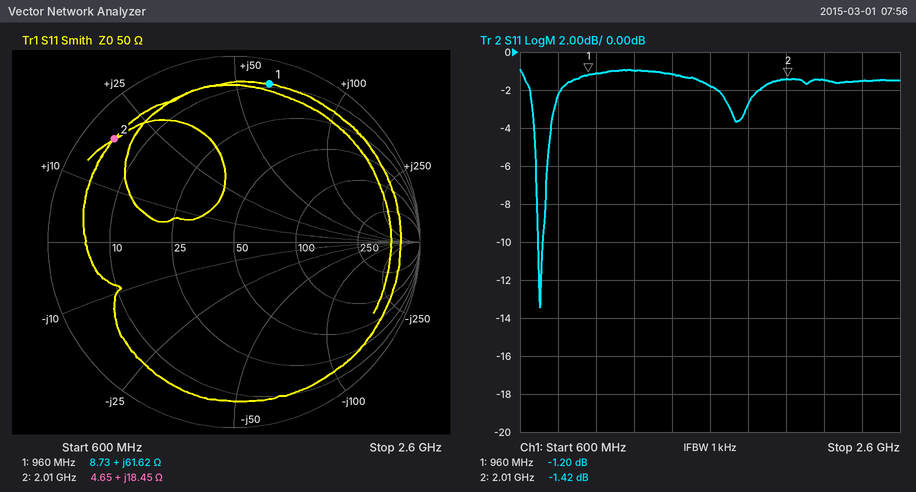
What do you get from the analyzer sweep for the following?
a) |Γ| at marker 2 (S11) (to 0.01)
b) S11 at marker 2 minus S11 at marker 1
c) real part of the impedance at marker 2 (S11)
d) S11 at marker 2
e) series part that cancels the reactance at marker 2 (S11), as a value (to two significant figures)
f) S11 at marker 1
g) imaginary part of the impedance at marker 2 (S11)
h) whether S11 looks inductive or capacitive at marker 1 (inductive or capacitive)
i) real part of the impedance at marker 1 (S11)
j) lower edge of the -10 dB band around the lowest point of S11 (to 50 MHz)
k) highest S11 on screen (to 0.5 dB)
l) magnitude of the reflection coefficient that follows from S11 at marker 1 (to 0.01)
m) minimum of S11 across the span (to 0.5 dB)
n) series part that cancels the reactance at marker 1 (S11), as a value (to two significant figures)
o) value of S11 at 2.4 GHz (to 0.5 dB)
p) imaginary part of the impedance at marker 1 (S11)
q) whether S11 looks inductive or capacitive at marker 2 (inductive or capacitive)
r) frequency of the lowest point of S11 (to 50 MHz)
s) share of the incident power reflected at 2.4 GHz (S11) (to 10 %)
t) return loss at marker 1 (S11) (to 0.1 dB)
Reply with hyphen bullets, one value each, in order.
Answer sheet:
- 0.85
- -0.22 dB
- 4.65 Ω
- -1.42 dB
- 4.3 pF
- -1.20 dB
- +18.45 Ω
- inductive
- 8.73 Ω
- 700 MHz
- -1.0 dB
- 0.87
- -13.5 dB
- 2.7 pF
- -1.5 dB
- +61.62 Ω
- inductive
- 700 MHz
- 70 %
- 1.2 dB
